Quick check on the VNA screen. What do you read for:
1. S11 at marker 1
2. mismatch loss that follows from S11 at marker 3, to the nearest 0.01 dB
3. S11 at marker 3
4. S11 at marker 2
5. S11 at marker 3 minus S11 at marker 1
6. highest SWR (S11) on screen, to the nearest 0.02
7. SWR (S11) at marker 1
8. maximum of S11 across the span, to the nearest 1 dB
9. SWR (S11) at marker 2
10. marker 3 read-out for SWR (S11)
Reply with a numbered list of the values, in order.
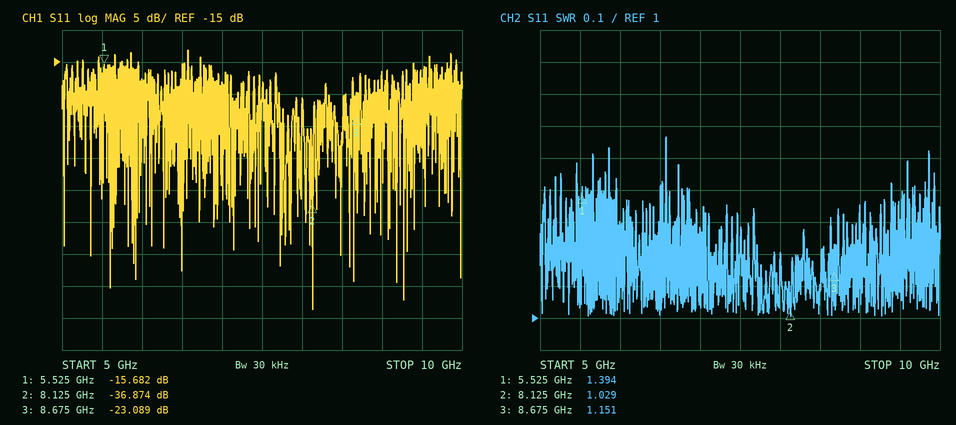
1. -15.682 dB
2. 0.02 dB
3. -23.089 dB
4. -36.874 dB
5. -7.407 dB
6. 1.56
7. 1.394
8. -13 dB
9. 1.029
10. 1.151
